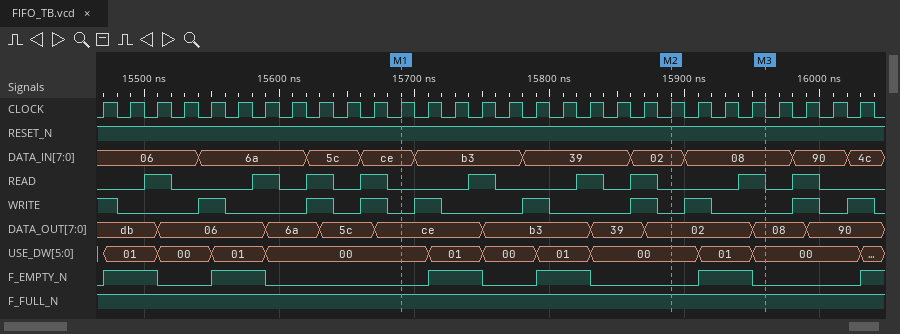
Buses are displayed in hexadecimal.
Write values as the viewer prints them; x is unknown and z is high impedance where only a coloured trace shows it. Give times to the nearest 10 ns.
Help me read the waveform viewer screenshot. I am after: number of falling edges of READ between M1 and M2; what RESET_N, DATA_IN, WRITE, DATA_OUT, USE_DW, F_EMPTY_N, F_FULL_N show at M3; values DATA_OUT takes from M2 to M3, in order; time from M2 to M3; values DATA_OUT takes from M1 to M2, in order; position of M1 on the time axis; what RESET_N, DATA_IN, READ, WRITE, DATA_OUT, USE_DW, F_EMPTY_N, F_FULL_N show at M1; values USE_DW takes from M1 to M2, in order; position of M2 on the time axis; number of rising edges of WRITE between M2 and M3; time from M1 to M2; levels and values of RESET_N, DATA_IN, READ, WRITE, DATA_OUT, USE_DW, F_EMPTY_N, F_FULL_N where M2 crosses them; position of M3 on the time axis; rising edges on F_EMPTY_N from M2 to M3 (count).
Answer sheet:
3
RESET_N=1, DATA_IN=08, WRITE=0, DATA_OUT=08, USE_DW=00, F_EMPTY_N=0, F_FULL_N=1
02, 08
70 ns
ce, b3, 39, 02
15690 ns
RESET_N=1, DATA_IN=ce, READ=0, WRITE=0, DATA_OUT=ce, USE_DW=00, F_EMPTY_N=0, F_FULL_N=1
00, 01, 00, 01, 00
15890 ns
1
200 ns
RESET_N=1, DATA_IN=02, READ=0, WRITE=0, DATA_OUT=02, USE_DW=00, F_EMPTY_N=0, F_FULL_N=1
15960 ns
1
